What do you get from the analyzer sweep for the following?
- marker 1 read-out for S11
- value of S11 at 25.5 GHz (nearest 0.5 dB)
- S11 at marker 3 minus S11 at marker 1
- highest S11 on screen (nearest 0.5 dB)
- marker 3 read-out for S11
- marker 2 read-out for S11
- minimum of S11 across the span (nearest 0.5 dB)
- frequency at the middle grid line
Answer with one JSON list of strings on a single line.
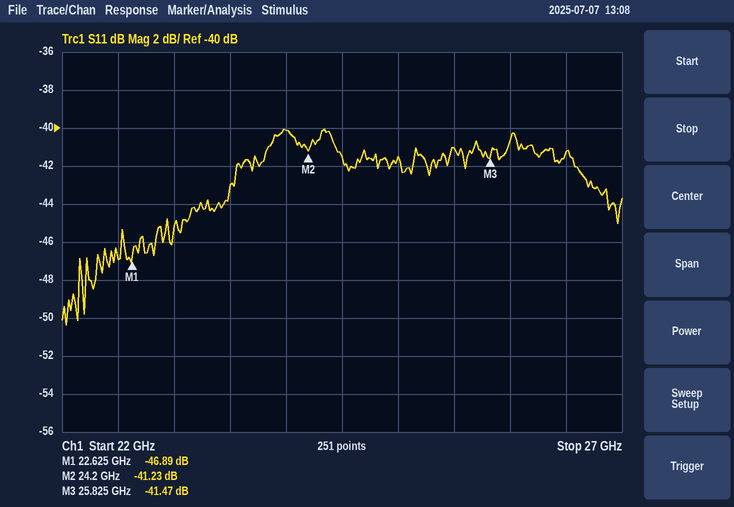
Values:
["-46.89 dB", "-41.0 dB", "5.42 dB", "-40.0 dB", "-41.47 dB", "-41.23 dB", "-50.5 dB", "24.5 GHz"]
